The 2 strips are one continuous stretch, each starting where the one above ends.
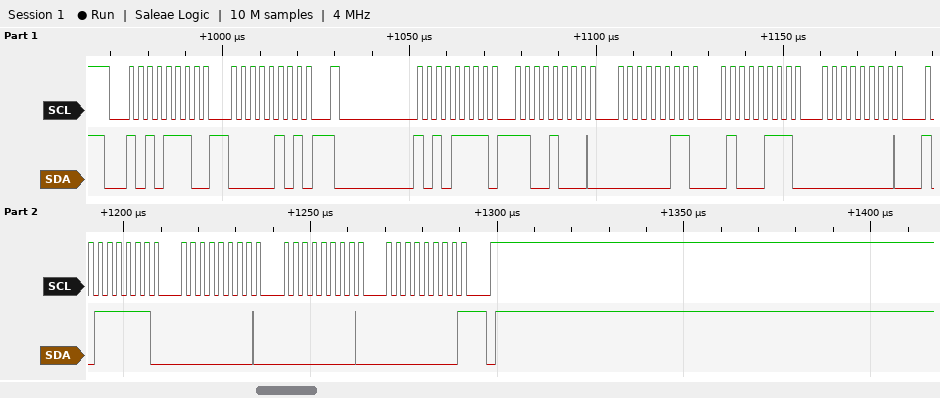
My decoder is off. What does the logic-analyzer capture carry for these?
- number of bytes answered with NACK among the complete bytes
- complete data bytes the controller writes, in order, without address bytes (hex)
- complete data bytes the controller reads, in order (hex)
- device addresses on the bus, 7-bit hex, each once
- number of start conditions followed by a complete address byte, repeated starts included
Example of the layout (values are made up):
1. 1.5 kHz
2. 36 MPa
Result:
1. 1
2. 05
3. C8 03 47 00 BF 00 00 00
4. 0x57
5. 2
